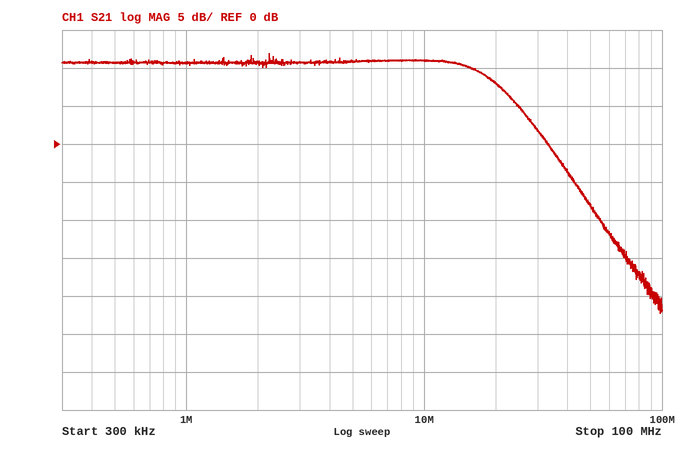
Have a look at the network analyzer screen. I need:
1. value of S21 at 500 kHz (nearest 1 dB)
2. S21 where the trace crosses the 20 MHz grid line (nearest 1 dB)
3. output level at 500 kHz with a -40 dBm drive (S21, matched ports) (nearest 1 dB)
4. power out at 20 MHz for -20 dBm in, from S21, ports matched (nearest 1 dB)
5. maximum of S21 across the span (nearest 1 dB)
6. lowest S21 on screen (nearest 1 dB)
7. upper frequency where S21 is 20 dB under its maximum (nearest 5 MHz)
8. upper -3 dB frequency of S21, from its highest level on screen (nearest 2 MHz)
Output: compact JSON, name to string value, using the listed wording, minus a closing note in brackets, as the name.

{"value of S21 at 500 kHz": "11 dB", "S21 where the trace crosses the 20 MHz grid line": "8 dB", "output level at 500 kHz with a -40 dBm drive (S21, matched ports)": "-29 dBm", "power out at 20 MHz for -20 dBm in, from S21, ports matched": "-12 dBm", "maximum of S21 across the span": "12 dB", "lowest S21 on screen": "-22 dB", "upper frequency where S21 is 20 dB under its maximum": "50 MHz", "upper -3 dB frequency of S21, from its highest level on screen": "18 MHz"}
